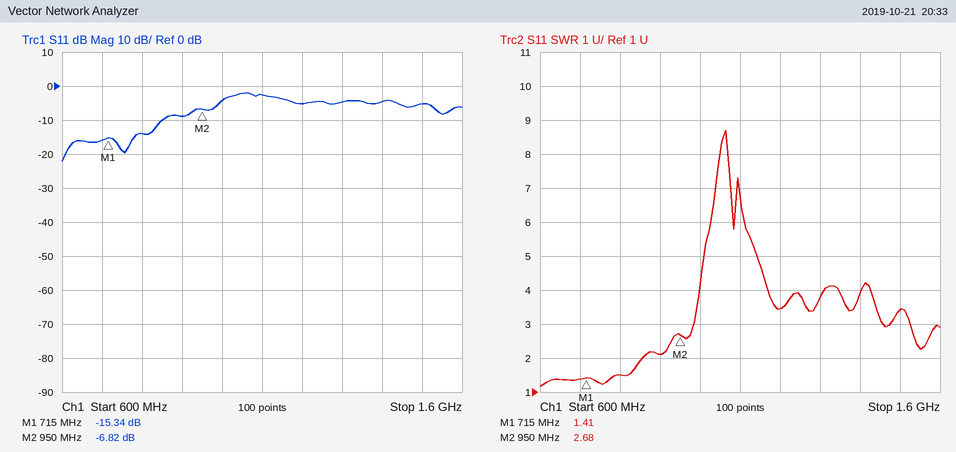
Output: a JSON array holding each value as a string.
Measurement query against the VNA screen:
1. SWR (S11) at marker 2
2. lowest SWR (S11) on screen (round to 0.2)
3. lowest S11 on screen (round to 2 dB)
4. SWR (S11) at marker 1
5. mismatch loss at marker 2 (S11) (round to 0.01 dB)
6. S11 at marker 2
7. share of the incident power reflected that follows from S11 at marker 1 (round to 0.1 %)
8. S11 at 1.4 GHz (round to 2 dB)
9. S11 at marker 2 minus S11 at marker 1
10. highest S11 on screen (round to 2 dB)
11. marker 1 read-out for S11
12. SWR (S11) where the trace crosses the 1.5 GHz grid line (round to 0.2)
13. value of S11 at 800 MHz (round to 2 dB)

["2.68", "1.2", "-22 dB", "1.41", "1.01 dB", "-6.82 dB", "2.9 %", "-4 dB", "8.52 dB", "-2 dB", "-15.34 dB", "3.4", "-14 dB"]
